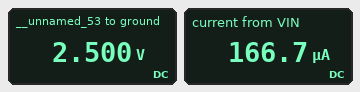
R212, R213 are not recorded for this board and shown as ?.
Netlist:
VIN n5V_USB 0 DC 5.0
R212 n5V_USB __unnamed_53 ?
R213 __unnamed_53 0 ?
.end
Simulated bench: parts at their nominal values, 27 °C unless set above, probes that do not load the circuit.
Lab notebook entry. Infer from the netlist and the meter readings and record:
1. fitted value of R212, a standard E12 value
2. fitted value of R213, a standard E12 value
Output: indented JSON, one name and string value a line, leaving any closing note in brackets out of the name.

{
  "fitted value of R212, a standard E12 value": "15 kΩ",
  "fitted value of R213, a standard E12 value": "15 kΩ"
}
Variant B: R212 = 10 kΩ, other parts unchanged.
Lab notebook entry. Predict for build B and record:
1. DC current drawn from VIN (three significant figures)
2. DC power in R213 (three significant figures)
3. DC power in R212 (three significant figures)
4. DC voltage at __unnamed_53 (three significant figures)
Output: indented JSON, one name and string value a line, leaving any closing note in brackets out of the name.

{
  "DC current drawn from VIN": "200 µA",
  "DC power in R213": "600 µW",
  "DC power in R212": "400 µW",
  "DC voltage at __unnamed_53": "3.00 V"
}
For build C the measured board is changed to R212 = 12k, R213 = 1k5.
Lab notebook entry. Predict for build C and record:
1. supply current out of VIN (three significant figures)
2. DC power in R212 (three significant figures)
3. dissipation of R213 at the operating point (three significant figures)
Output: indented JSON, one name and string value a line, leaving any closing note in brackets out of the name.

{
  "supply current out of VIN": "370 µA",
  "DC power in R212": "1.65 mW",
  "dissipation of R213 at the operating point": "206 µW"
}
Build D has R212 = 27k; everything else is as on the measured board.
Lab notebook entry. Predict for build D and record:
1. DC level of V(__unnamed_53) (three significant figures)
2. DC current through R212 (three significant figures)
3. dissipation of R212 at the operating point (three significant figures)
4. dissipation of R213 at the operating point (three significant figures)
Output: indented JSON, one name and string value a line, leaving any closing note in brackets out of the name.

{
  "DC level of V(__unnamed_53)": "1.79 V",
  "DC current through R212": "119 µA",
  "dissipation of R212 at the operating point": "383 µW",
  "dissipation of R213 at the operating point": "213 µW"
}
